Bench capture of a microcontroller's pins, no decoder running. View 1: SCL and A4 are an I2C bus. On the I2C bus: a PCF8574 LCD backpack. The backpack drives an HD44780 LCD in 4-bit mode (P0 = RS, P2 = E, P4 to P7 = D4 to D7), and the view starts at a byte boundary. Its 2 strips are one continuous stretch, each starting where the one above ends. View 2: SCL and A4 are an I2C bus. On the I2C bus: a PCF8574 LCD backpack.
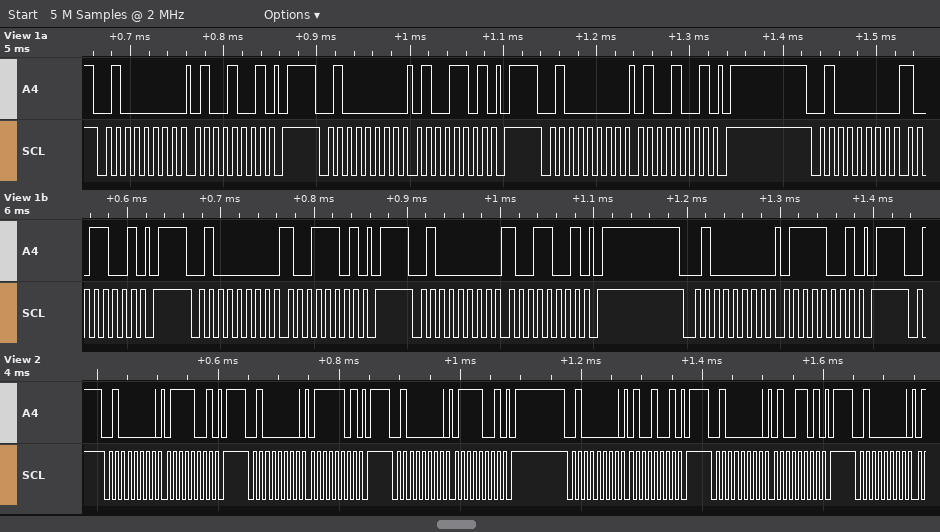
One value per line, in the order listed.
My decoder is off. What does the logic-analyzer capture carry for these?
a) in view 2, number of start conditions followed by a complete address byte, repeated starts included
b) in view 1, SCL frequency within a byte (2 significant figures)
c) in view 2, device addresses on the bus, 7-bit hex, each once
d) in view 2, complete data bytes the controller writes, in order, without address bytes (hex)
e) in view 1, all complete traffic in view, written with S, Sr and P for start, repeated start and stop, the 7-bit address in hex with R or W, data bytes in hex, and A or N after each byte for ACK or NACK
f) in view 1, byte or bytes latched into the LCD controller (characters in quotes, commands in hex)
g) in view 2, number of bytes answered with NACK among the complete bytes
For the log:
6
100 kHz
0x20
79 7D 79 49 4D
S 20W A 49 A P S 20W A 4D A P S 20W A 49 A P S 20W A 99 A P S 20W A 9D A P S 20W A 99 A P S 20W A 79 A P
'I'
0
